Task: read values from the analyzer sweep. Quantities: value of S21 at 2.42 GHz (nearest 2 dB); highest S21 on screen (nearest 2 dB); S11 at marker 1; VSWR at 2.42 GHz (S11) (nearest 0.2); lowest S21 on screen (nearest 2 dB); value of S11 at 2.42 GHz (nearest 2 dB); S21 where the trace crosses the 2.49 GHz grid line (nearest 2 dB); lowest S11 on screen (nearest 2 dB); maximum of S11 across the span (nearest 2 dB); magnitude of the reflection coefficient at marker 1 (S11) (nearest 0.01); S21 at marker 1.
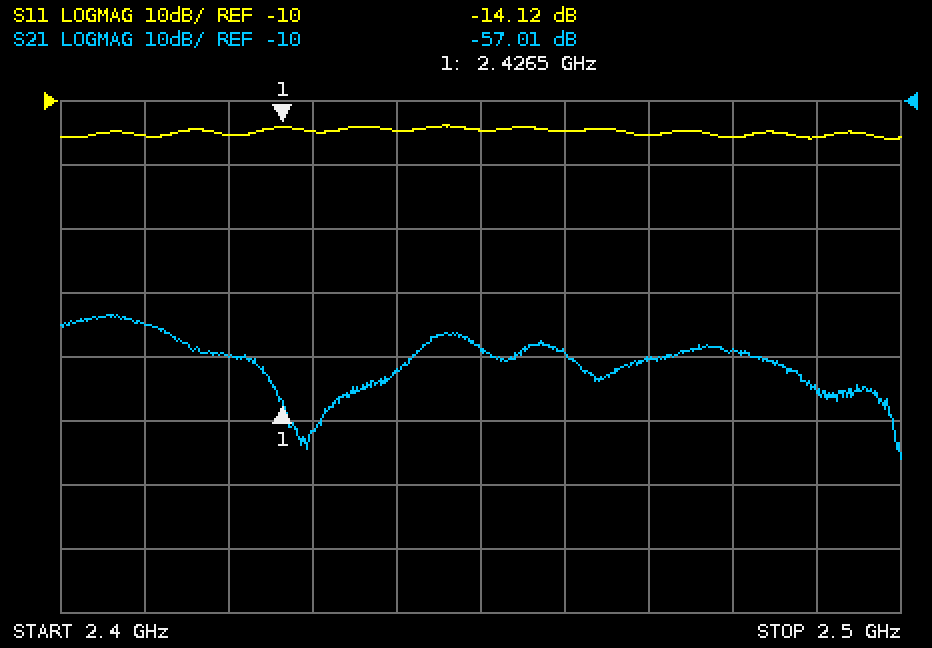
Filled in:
-50 dB
-44 dB
-14.12 dB
1.4
-66 dB
-16 dB
-56 dB
-16 dB
-14 dB
0.20
-57.01 dB
